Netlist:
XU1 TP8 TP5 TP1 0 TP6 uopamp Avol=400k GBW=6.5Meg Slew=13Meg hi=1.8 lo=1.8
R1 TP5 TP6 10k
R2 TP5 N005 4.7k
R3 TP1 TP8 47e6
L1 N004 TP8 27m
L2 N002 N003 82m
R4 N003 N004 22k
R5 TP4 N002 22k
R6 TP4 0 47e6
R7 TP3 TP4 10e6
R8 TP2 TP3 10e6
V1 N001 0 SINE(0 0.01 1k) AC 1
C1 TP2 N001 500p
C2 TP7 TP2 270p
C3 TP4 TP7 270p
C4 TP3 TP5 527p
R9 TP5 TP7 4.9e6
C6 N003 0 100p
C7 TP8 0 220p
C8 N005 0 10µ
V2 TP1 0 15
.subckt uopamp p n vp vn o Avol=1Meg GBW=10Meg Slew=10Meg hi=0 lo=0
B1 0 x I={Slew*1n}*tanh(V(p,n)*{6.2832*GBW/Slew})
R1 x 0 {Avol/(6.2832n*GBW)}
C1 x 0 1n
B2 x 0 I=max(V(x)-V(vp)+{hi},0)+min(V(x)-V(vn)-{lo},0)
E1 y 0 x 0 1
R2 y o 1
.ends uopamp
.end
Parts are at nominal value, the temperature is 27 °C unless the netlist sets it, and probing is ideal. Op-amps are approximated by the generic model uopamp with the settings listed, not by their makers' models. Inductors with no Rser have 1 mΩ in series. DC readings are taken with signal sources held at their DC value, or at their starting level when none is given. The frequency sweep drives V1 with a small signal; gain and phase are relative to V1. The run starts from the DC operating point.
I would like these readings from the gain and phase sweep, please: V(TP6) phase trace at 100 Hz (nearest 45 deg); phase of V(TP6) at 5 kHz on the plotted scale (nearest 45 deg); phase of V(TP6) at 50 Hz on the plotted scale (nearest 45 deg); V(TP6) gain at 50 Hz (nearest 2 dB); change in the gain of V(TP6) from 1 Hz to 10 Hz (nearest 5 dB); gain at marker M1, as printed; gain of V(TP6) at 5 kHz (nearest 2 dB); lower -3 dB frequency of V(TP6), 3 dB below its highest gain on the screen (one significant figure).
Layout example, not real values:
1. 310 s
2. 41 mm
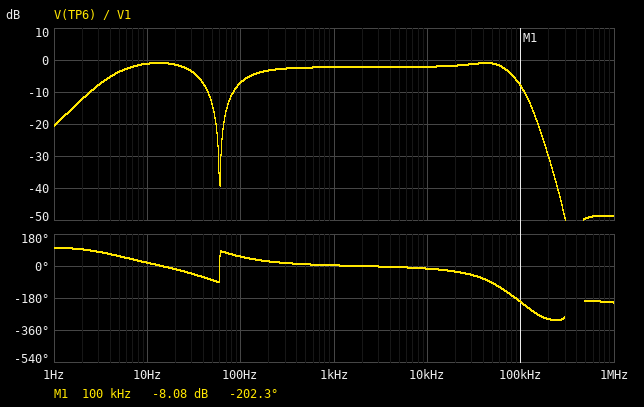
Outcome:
1. 45 deg
2. 0 deg
3. -90 deg
4. -14 dB
5. 20 dB
6. -8.08 dB
7. -2 dB
8. 5 Hz
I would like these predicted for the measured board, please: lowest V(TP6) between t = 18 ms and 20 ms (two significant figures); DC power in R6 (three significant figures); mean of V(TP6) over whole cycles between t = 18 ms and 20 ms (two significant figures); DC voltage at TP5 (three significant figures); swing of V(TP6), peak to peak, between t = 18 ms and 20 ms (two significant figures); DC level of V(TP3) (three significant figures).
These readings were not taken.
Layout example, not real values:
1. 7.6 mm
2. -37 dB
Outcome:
1. 7.5 V
2. 1.20 µW
3. 7.5 V
4. 7.50 V
5. 15 mV
6. 7.50 V
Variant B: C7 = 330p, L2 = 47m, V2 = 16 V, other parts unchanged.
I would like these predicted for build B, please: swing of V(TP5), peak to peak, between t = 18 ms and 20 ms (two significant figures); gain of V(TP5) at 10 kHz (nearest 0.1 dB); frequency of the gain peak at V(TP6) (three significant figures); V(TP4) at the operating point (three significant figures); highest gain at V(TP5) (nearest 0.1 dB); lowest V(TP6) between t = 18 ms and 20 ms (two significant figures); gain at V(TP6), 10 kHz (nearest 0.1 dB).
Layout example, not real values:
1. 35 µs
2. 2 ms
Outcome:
1. 3.9 mV
2. -14.1 dB
3. 12.0 Hz
4. 8.00 V
5. -11.1 dB
6. 8.0 V
7. -4.2 dB
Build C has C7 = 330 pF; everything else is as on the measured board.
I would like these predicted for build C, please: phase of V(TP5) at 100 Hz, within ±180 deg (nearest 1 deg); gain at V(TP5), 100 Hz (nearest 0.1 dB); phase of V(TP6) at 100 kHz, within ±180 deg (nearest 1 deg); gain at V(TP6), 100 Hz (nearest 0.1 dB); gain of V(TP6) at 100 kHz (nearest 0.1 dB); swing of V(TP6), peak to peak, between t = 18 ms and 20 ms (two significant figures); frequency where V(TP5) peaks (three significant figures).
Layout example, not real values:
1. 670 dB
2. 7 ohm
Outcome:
1. 50 deg
2. -19.3 dB
3. 154 deg
4. -9.4 dB
5. -11.3 dB
6. 12 mV
7. 10.7 Hz
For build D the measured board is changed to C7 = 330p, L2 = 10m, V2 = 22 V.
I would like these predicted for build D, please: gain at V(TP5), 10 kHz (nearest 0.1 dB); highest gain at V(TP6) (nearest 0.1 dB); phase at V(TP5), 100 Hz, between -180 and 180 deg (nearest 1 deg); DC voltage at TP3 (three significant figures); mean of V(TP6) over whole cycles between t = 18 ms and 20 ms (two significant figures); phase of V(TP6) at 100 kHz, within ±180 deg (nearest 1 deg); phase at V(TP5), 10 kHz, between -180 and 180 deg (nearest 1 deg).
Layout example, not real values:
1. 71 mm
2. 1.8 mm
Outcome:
1. -14.2 dB
2. -1.5 dB
3. 50 deg
4. 11.0 V
5. 11 V
6. -139 deg
7. -16 deg
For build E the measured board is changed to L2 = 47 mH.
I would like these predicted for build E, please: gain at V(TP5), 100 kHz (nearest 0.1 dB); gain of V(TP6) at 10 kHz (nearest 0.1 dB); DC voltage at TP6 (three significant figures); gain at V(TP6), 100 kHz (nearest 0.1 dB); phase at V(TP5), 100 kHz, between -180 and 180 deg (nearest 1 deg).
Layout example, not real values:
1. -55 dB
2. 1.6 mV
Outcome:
1. -16.3 dB
2. -2.2 dB
3. 7.50 V
4. -6.3 dB
5. -170 deg
